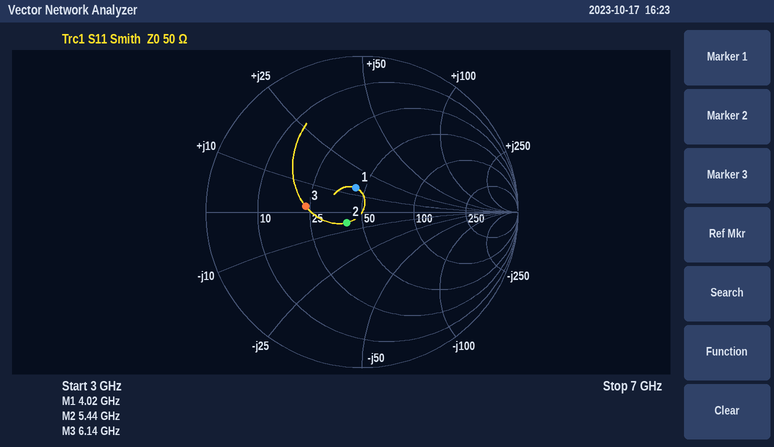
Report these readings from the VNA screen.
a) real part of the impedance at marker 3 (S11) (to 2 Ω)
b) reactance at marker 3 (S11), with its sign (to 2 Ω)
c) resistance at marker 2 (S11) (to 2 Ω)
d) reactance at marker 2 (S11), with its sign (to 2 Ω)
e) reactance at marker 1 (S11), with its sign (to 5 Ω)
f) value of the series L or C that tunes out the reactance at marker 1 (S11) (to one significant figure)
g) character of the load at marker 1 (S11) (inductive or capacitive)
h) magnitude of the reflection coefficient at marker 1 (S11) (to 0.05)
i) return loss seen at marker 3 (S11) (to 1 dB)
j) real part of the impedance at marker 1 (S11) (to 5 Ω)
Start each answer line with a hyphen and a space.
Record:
- 24 Ω
- +2 Ω
- 40 Ω
- -6 Ω
- +15 Ω
- 3 pF
- inductive
- 0.15
- 9 dB
- 45 Ω
